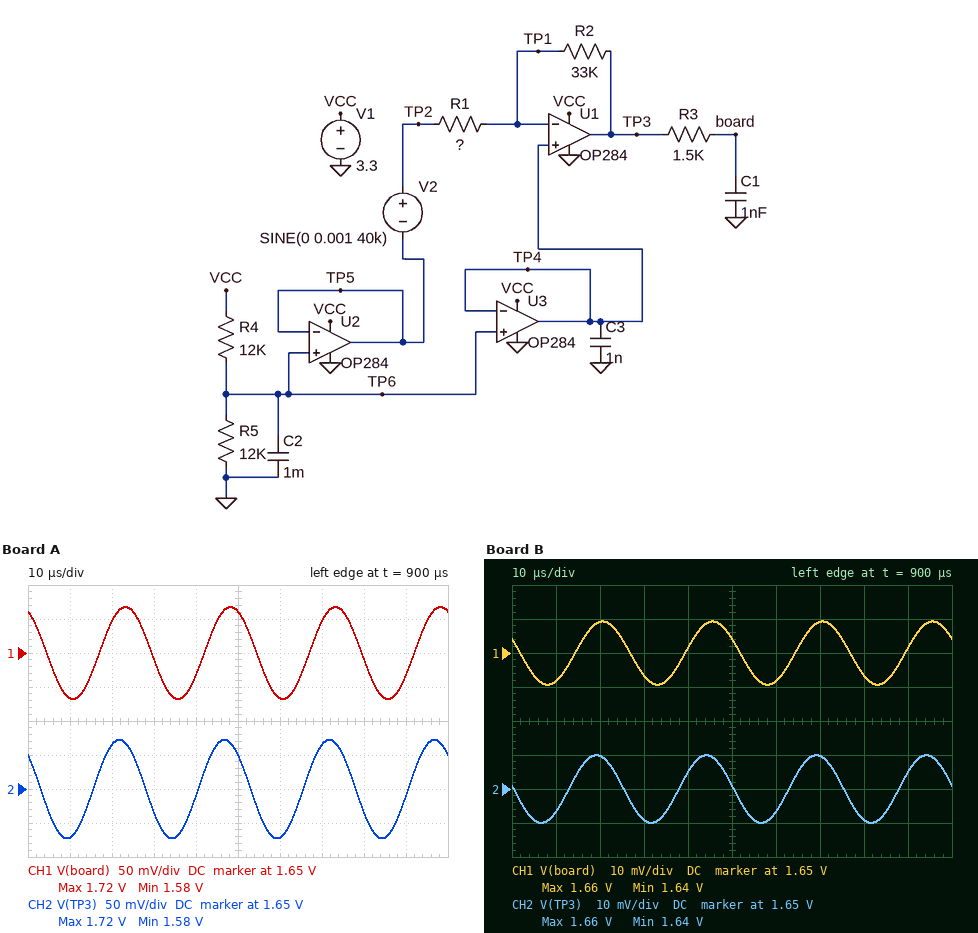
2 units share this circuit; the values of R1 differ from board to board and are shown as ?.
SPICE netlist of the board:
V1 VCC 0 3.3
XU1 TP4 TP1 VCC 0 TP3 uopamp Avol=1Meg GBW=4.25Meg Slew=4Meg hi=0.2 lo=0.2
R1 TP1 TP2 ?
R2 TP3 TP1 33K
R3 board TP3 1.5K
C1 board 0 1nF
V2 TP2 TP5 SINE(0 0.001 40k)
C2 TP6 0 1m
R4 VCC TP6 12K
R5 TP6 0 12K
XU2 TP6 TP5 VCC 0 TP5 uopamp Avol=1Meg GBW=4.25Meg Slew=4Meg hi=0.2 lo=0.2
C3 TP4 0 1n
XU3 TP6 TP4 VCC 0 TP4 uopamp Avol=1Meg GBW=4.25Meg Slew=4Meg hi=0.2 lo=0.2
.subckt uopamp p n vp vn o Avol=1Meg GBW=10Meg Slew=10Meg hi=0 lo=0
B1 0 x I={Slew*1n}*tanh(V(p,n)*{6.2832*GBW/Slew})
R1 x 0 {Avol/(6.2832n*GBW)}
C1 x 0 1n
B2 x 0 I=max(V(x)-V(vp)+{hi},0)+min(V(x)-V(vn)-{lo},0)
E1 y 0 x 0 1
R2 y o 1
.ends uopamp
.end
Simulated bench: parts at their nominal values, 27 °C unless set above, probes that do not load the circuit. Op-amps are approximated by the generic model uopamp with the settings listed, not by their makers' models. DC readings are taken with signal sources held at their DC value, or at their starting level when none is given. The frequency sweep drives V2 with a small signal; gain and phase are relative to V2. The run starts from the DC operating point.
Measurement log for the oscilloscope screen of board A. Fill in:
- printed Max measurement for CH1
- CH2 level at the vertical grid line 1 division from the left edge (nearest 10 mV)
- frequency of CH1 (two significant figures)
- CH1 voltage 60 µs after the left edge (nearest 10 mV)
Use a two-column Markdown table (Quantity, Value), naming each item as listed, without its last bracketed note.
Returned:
| Quantity | Value |
|---|---|
| printed Max measurement for CH1 | 1.72 V |
| CH2 level at the vertical grid line 1 division from the left edge | 1.58 V |
| frequency of CH1 | 40 kHz |
| CH1 voltage 60 µs after the left edge | 1.58 V |
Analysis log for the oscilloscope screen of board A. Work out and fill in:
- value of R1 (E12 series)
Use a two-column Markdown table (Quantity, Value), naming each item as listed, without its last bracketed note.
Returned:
| Quantity | Value |
|---|---|
| value of R1 | 330 Ω |
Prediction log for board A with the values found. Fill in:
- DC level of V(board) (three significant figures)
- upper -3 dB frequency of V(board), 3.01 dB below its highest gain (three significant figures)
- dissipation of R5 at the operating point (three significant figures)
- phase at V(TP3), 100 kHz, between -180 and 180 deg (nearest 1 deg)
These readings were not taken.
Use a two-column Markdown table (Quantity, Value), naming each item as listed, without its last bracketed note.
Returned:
| Quantity | Value |
|---|---|
| DC level of V(board) | 1.65 V |
| upper -3 dB frequency of V(board), 3.01 dB below its highest gain | 37.2 kHz |
| dissipation of R5 at the operating point | 227 µW |
| phase at V(TP3), 100 kHz, between -180 and 180 deg | 113 deg |
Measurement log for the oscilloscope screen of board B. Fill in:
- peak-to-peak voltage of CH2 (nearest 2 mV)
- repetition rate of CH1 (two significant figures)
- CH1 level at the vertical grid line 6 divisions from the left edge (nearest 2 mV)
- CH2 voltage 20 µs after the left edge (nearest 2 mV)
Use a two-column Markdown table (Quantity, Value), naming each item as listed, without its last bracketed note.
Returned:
| Quantity | Value |
|---|---|
| peak-to-peak voltage of CH2 | 20 mV |
| repetition rate of CH1 | 40 kHz |
| CH1 level at the vertical grid line 6 divisions from the left edge | 1.642 V |
| CH2 voltage 20 µs after the left edge | 1.660 V |
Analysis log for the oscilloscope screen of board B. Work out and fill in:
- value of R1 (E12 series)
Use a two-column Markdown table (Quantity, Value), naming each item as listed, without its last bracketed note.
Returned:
| Quantity | Value |
|---|---|
| value of R1 | 3.3 kΩ |
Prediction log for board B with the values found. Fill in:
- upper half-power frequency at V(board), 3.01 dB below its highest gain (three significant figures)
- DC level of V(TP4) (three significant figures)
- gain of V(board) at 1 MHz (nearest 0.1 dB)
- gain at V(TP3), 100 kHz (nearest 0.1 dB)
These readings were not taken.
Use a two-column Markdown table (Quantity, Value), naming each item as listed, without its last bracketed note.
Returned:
| Quantity | Value |
|---|---|
| upper half-power frequency at V(board), 3.01 dB below its highest gain | 99.3 kHz |
| DC level of V(TP4) | 1.65 V |
| gain of V(board) at 1 MHz | -8.4 dB |
| gain at V(TP3), 100 kHz | 19.7 dB |
